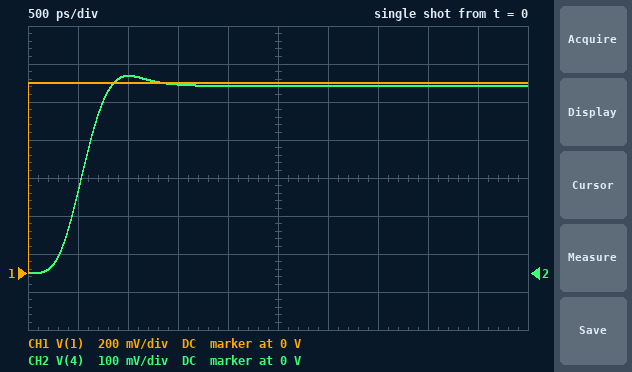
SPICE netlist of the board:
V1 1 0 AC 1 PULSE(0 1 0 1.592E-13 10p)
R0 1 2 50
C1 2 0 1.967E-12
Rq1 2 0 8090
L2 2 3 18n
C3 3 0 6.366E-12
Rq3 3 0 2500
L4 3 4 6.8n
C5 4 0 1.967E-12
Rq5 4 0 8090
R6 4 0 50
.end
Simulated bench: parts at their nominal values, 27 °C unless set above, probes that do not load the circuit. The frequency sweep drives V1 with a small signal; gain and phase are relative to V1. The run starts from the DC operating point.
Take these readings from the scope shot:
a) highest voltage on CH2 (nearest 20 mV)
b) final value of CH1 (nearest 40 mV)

520 mV
1.00 V
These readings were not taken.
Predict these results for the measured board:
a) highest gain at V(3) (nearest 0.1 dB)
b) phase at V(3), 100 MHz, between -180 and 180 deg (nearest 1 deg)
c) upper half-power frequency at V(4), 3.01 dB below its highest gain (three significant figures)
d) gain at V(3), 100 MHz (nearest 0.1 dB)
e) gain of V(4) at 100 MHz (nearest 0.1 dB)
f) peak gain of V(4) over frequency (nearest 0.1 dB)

-6.2 dB
-13 deg
842 MHz
-6.2 dB
-6.2 dB
-6.2 dB
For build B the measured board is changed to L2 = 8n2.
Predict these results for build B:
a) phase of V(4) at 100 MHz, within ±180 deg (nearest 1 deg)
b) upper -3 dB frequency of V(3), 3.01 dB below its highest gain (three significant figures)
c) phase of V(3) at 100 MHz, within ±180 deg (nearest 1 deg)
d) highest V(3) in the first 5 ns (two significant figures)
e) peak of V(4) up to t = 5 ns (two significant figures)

-15 deg
1.53 GHz
-10 deg
520 mV
540 mV
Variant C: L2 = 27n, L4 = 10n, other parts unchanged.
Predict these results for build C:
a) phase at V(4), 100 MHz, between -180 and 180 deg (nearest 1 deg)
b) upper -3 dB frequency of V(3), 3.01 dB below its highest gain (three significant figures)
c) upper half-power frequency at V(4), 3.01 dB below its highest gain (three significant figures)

-23 deg
742 MHz
678 MHz
